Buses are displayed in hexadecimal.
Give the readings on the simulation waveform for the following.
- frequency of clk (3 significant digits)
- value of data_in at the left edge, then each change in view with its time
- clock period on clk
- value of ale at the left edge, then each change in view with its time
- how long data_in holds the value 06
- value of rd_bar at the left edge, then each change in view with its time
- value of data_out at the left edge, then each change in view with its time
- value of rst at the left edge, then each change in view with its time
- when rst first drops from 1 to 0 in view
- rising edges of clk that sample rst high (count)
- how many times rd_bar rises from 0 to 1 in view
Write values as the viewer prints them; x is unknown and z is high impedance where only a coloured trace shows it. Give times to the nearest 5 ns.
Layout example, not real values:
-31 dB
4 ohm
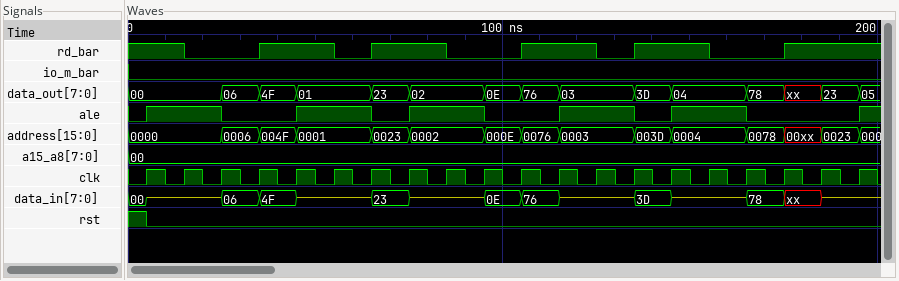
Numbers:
100 MHz
00, z at 5 ns, 06 at 25 ns, 4F at 35 ns, z at 45 ns, 23 at 65 ns, z at 75 ns, 0E at 95 ns, 76 at 105 ns, z at 115 ns, 3D at 135 ns, z at 145 ns, 78 at 165 ns, xx at 175 ns, z at 185 ns
10 ns
0, 1 at 5 ns, 0 at 25 ns, 1 at 45 ns, 0 at 65 ns, 1 at 75 ns, 0 at 95 ns, 1 at 115 ns, 0 at 135 ns, 1 at 145 ns, 0 at 165 ns, 1 at 195 ns
10 ns
1, 0 at 15 ns, 1 at 35 ns, 0 at 55 ns, 1 at 65 ns, 0 at 85 ns, 1 at 105 ns, 0 at 125 ns, 1 at 135 ns, 0 at 155 ns, 1 at 175 ns
00, 06 at 25 ns, 4F at 35 ns, 01 at 45 ns, 23 at 65 ns, 02 at 75 ns, 0E at 95 ns, 76 at 105 ns, 03 at 115 ns, 3D at 135 ns, 04 at 145 ns, 78 at 165 ns, xx at 175 ns, 23 at 185 ns, 05 at 195 ns
1, 0 at 5 ns
5 ns
1
5
